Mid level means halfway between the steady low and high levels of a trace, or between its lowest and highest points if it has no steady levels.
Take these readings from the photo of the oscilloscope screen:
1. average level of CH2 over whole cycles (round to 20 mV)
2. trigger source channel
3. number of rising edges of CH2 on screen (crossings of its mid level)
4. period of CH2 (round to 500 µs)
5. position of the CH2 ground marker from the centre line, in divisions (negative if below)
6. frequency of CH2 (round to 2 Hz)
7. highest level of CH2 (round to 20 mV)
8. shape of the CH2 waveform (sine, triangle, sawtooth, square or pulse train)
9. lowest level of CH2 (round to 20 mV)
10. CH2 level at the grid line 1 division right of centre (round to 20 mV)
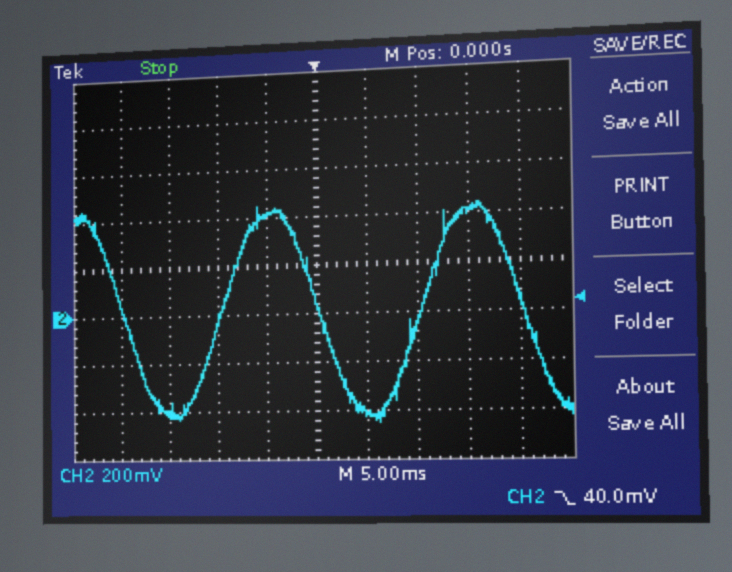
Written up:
0 mV
CH2
2
20.0 ms
-1.0 div
50 Hz
440 mV
sine
-440 mV
-400 mV
